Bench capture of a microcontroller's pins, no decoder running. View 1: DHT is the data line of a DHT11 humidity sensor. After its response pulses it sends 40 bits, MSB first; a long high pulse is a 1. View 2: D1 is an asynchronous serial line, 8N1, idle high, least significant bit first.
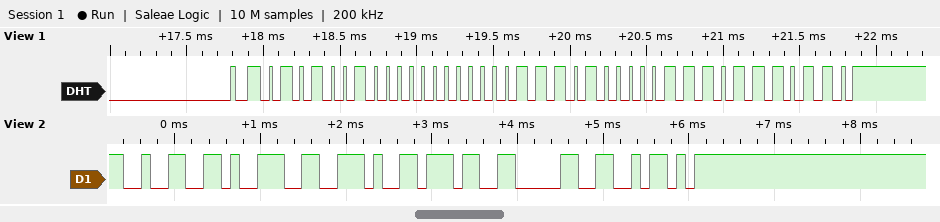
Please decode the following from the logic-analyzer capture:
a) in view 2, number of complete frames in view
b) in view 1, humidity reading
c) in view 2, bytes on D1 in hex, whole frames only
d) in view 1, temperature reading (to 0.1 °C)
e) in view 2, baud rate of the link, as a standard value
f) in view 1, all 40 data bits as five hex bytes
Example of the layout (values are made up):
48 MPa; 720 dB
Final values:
6; 82 %; 32 39 2E 37 30 5A; 29.7 °C; 9600 baud; 52 00 1D 07 76
